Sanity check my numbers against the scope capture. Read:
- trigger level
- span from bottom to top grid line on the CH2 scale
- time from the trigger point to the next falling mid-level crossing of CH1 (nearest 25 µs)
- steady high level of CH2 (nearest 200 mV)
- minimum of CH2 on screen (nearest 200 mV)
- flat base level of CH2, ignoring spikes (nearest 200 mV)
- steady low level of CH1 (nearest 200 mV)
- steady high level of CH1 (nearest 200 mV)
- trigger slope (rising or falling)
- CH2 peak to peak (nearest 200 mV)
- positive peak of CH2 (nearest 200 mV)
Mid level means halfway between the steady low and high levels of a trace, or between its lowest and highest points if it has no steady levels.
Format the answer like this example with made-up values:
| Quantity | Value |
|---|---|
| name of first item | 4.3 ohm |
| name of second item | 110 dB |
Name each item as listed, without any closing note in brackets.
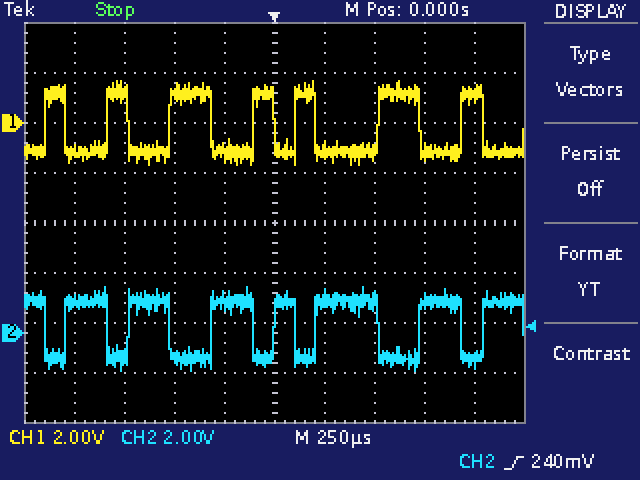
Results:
| Quantity | Value |
|---|---|
| trigger level | 240 mV |
| span from bottom to top grid line on the CH2 scale | 16 V |
| time from the trigger point to the next falling mid-level crossing of CH1 | 200 µs |
| steady high level of CH2 | 1.2 V |
| minimum of CH2 on screen | -1.6 V |
| flat base level of CH2, ignoring spikes | -1.0 V |
| steady low level of CH1 | -1.2 V |
| steady high level of CH1 | 1.2 V |
| trigger slope | rising |
| CH2 peak to peak | 3.4 V |
| positive peak of CH2 | 1.8 V |
